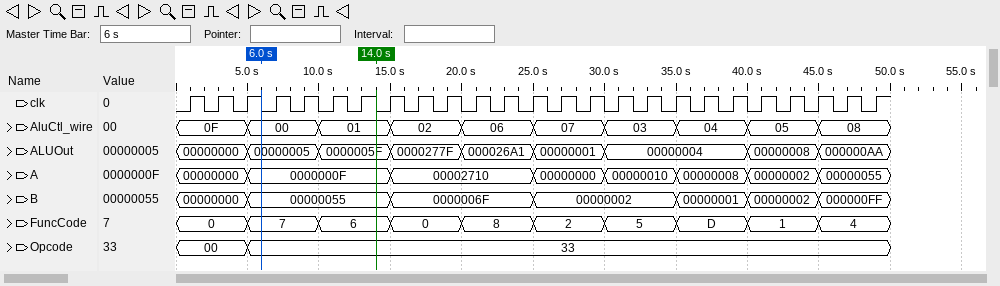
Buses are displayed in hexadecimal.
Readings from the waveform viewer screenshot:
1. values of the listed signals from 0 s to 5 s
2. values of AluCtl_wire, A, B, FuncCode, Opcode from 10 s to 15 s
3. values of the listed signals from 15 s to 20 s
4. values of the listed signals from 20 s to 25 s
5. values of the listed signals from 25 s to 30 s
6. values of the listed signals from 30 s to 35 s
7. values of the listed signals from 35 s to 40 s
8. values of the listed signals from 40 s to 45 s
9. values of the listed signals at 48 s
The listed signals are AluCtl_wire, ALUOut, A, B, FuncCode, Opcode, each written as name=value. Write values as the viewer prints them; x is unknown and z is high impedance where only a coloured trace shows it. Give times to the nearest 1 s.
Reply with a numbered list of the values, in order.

1. AluCtl_wire=0F, ALUOut=00000000, A=00000000, B=00000000, FuncCode=0, Opcode=00
2. AluCtl_wire=01, A=0000000F, B=00000055, FuncCode=6, Opcode=33
3. AluCtl_wire=02, ALUOut=0000277F, A=00002710, B=0000006F, FuncCode=0, Opcode=33
4. AluCtl_wire=06, ALUOut=000026A1, A=00002710, B=0000006F, FuncCode=8, Opcode=33
5. AluCtl_wire=07, ALUOut=00000001, A=00000000, B=00000002, FuncCode=2, Opcode=33
6. AluCtl_wire=03, ALUOut=00000004, A=00000010, B=00000002, FuncCode=5, Opcode=33
7. AluCtl_wire=04, ALUOut=00000004, A=00000008, B=00000001, FuncCode=D, Opcode=33
8. AluCtl_wire=05, ALUOut=00000008, A=00000002, B=00000002, FuncCode=1, Opcode=33
9. AluCtl_wire=08, ALUOut=000000AA, A=00000055, B=000000FF, FuncCode=4, Opcode=33
